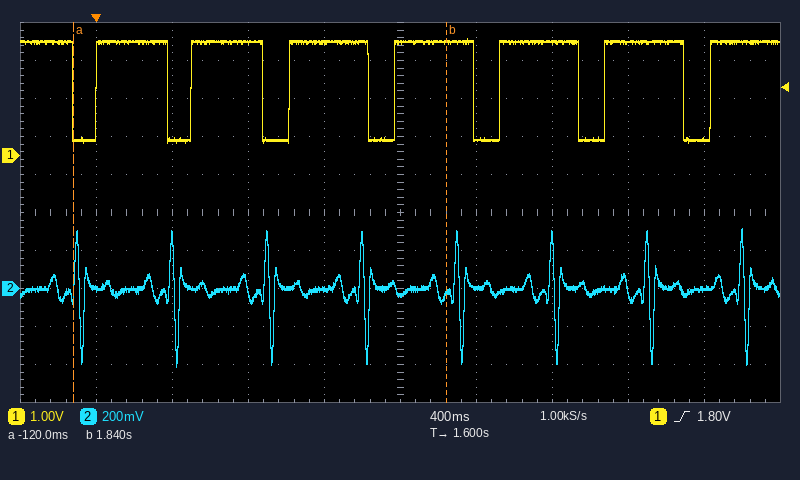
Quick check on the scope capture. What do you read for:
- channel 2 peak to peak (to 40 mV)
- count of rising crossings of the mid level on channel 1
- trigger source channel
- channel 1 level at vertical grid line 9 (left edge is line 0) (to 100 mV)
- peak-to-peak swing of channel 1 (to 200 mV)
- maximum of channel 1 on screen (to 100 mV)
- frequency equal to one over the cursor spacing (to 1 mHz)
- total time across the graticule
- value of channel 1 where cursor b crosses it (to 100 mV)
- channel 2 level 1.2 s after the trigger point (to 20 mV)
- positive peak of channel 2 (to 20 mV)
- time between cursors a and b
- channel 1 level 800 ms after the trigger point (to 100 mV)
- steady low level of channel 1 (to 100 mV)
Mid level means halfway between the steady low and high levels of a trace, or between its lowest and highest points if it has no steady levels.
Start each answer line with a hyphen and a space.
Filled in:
- 720 mV
- 7
- channel 1
- 400 mV
- 2.8 V
- 3.1 V
- 510 mHz
- 4 s
- 3.0 V
- 0 mV
- 320 mV
- 1.96 s
- 3.0 V
- 400 mV
